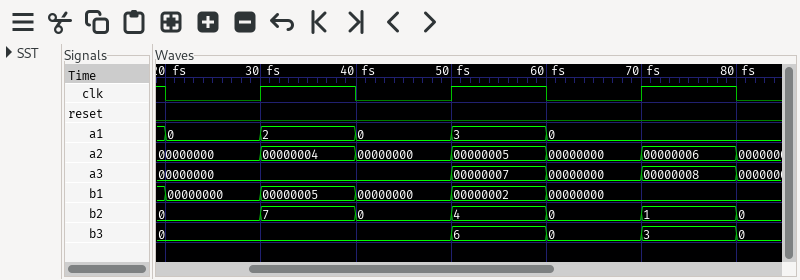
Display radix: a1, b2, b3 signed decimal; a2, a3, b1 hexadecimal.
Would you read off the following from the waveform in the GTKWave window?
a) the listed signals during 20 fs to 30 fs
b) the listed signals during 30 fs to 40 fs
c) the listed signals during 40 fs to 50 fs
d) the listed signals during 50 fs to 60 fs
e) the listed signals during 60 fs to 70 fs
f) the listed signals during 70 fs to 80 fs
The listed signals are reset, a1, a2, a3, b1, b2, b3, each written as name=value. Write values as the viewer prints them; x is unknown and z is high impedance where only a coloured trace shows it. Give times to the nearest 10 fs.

reset=0, a1=0, a2=00000000, a3=00000000, b1=00000000, b2=0, b3=0
reset=0, a1=2, a2=00000004, a3=00000000, b1=00000005, b2=7, b3=0
reset=0, a1=0, a2=00000000, a3=00000000, b1=00000000, b2=0, b3=0
reset=0, a1=3, a2=00000005, a3=00000007, b1=00000002, b2=4, b3=6
reset=0, a1=0, a2=00000000, a3=00000000, b1=00000000, b2=0, b3=0
reset=0, a1=0, a2=00000006, a3=00000008, b1=00000000, b2=1, b3=3
